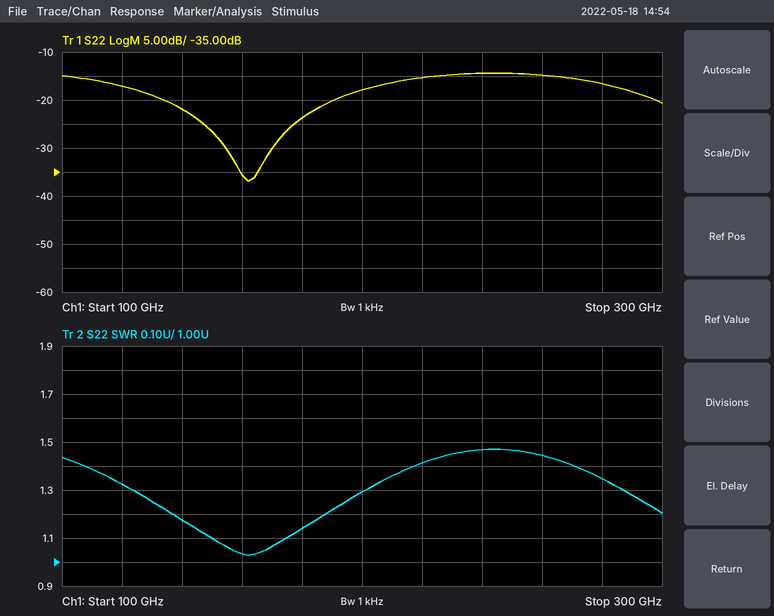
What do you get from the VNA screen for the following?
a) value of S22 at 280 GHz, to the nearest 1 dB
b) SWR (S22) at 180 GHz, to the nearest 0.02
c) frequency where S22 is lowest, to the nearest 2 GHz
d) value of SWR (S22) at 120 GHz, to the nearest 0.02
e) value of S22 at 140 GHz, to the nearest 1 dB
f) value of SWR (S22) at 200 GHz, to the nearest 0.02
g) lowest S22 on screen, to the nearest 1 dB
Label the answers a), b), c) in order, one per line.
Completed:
a) -17 dB
b) 1.14
c) 162 GHz
d) 1.32
e) -22 dB
f) 1.30
g) -37 dB
